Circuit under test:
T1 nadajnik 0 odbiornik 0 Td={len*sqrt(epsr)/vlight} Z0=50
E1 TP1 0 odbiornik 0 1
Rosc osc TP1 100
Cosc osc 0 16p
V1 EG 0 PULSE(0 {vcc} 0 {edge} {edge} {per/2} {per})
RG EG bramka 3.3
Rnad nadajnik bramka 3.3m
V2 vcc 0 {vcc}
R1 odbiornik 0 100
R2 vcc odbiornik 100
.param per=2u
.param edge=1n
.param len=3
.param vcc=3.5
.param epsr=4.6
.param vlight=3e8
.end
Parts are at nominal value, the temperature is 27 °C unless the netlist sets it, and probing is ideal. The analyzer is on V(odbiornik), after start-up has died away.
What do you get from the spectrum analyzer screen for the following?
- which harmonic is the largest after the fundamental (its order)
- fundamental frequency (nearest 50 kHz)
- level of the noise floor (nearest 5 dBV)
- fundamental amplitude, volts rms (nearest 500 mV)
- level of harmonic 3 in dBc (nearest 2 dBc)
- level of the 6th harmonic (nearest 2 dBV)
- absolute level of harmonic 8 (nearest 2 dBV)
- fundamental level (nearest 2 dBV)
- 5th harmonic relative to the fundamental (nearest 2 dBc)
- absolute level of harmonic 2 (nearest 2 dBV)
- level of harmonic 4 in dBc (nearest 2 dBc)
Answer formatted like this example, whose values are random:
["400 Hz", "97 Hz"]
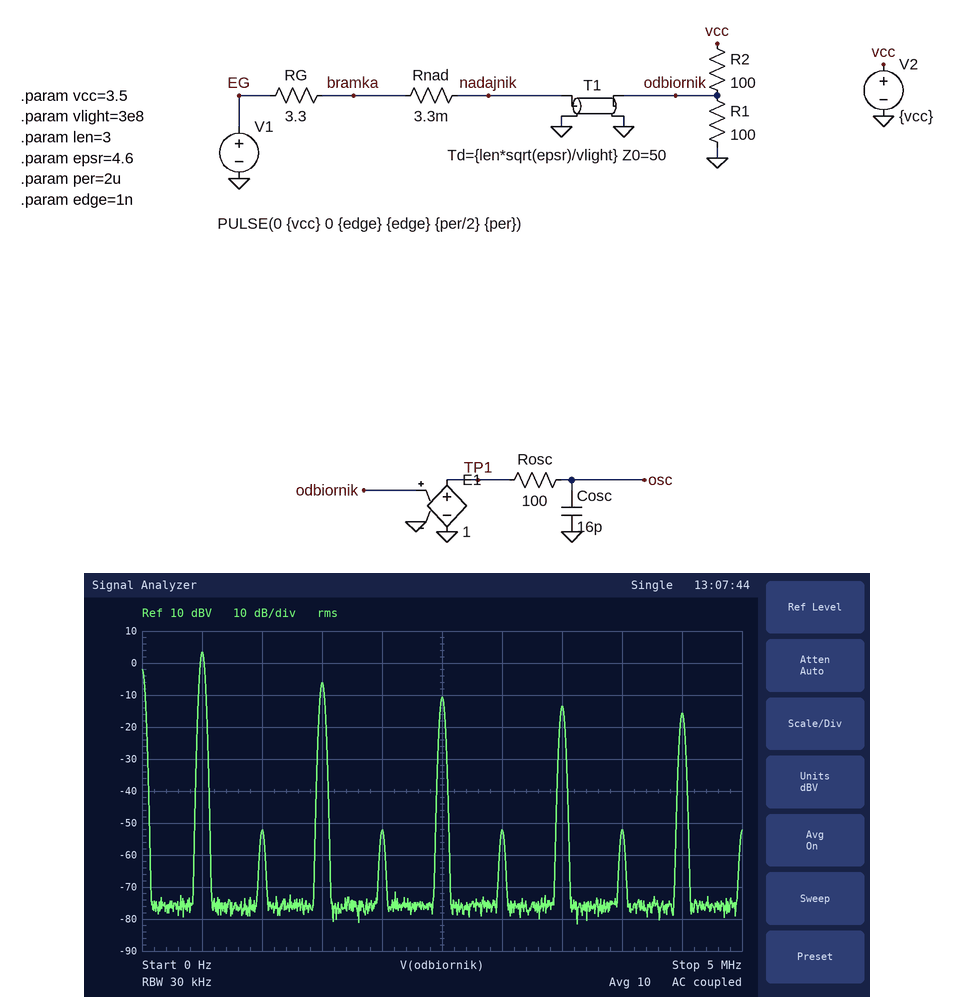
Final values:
["3", "500 kHz", "-75 dBV", "1.5 V", "-10 dBc", "-52 dBV", "-52 dBV", "4 dBV", "-14 dBc", "-52 dBV", "-56 dBc"]
